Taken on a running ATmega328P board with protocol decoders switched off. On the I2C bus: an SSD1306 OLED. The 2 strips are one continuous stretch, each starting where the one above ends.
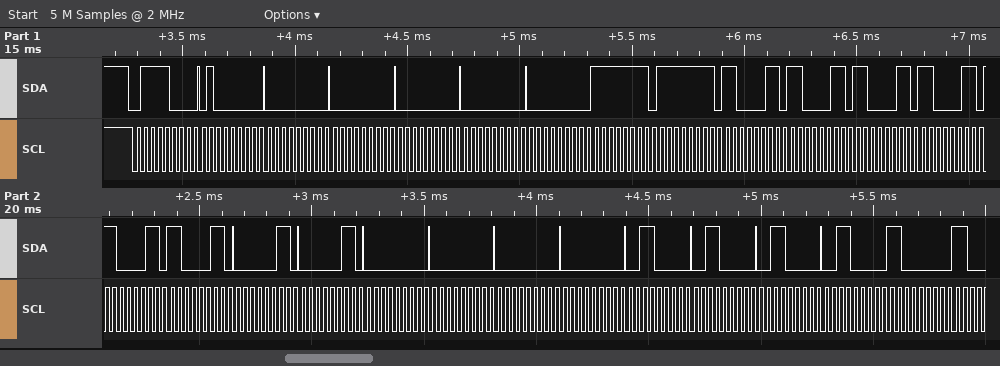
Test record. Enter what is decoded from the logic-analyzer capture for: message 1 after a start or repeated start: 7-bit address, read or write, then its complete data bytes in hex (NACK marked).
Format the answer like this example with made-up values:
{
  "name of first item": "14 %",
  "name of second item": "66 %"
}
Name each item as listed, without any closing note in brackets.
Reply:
{
  "message 1 after a start or repeated start: 7-bit address, read or write, then its complete data bytes in hex": "0x3C write: 40 00 00 00 00 00 FF FF C3 C3 C3 C3 C3 C3 03 03 00 00 00 00 30 30 30 30 C0"
}
